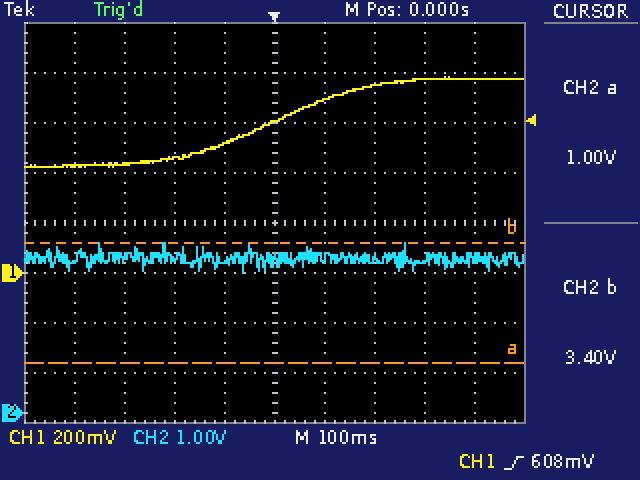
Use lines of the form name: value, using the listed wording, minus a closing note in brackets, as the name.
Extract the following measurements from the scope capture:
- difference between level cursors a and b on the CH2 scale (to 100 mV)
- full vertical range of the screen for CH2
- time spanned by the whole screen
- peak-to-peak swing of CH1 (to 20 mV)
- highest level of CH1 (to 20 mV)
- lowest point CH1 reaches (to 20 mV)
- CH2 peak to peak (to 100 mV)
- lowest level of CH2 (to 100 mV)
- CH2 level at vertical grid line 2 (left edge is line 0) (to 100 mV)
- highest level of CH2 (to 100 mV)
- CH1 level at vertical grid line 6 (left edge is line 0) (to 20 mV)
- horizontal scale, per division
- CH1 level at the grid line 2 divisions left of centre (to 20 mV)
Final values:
difference between level cursors a and b on the CH2 scale: 2.4 V
full vertical range of the screen for CH2: 8 V
time spanned by the whole screen: 1 s
peak-to-peak swing of CH1: 360 mV
highest level of CH1: 780 mV
lowest point CH1 reaches: 420 mV
CH2 peak to peak: 600 mV
lowest level of CH2: 2.8 V
CH2 level at vertical grid line 2 (left edge is line 0): 3.1 V
highest level of CH2: 3.4 V
CH1 level at vertical grid line 6 (left edge is line 0): 700 mV
horizontal scale, per division: 100 ms
CH1 level at the grid line 2 divisions left of centre: 460 mV
